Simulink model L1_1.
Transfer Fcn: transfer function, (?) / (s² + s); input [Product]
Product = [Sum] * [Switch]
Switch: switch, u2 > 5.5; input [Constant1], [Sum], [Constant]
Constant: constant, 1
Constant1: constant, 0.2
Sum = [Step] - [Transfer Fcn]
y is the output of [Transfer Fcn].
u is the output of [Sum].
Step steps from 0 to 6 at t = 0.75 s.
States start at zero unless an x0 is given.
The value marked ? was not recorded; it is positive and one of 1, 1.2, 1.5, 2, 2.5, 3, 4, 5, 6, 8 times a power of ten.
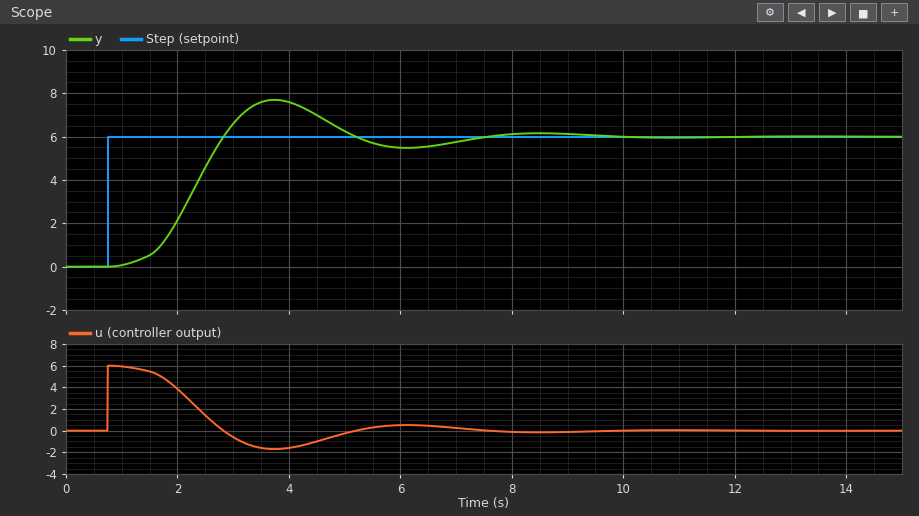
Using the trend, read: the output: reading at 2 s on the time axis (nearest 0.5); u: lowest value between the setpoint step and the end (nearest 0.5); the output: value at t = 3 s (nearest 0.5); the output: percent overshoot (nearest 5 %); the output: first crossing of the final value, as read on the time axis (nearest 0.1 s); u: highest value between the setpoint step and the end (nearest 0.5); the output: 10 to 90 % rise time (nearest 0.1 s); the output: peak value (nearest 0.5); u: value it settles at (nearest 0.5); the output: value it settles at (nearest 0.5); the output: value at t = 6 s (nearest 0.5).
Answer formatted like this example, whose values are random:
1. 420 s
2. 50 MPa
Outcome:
1. 2.0
2. -1.5
3. 6.5
4. 30 %
5. 2.8 s
6. 6.0
7. 1.1 s
8. 7.5
9. 0.0
10. 6.0
11. 5.5
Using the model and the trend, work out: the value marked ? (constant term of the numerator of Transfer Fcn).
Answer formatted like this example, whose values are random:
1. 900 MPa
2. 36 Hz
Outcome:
1. 2
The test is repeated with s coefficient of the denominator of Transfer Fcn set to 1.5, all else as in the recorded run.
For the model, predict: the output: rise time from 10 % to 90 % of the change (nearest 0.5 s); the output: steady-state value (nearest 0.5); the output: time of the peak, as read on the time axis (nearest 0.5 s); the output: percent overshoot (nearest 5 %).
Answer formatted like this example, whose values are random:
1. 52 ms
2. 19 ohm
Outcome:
1. 1.5 s
2. 6.0
3. 4.0 s
4. 15 %
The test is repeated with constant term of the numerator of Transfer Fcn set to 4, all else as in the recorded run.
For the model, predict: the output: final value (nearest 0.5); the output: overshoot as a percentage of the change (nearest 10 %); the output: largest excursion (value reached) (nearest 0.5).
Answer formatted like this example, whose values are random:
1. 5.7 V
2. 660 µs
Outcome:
1. 6.0
2. 40 %
3. 8.5
